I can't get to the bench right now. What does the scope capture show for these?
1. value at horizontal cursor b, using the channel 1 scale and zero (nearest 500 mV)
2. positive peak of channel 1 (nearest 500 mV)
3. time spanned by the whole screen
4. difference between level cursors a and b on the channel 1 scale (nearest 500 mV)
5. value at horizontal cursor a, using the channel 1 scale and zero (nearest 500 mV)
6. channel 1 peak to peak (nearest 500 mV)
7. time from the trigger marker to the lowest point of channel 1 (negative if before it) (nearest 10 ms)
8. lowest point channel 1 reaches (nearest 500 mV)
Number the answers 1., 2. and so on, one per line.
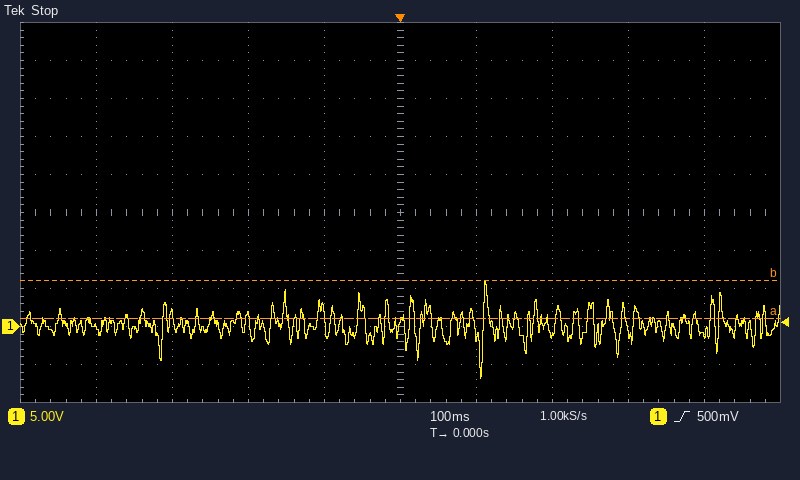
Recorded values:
1. 6.0 V
2. 6.0 V
3. 1 s
4. 5.0 V
5. 1.0 V
6. 13.0 V
7. +110 ms
8. -7.0 V
